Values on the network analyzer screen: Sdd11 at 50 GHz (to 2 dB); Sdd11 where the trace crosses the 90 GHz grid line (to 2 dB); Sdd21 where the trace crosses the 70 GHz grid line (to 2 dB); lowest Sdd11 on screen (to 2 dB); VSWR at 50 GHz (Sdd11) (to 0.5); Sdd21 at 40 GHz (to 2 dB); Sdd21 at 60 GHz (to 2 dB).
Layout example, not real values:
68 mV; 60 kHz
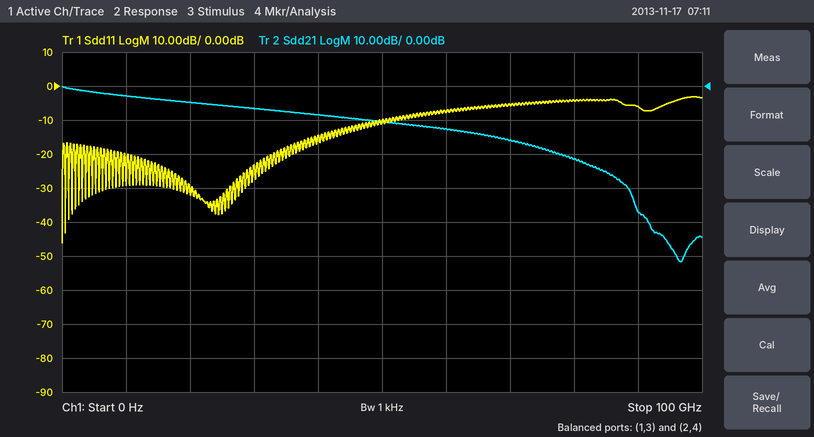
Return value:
-10 dB; -6 dB; -16 dB; -46 dB; 2.0; -8 dB; -12 dB
